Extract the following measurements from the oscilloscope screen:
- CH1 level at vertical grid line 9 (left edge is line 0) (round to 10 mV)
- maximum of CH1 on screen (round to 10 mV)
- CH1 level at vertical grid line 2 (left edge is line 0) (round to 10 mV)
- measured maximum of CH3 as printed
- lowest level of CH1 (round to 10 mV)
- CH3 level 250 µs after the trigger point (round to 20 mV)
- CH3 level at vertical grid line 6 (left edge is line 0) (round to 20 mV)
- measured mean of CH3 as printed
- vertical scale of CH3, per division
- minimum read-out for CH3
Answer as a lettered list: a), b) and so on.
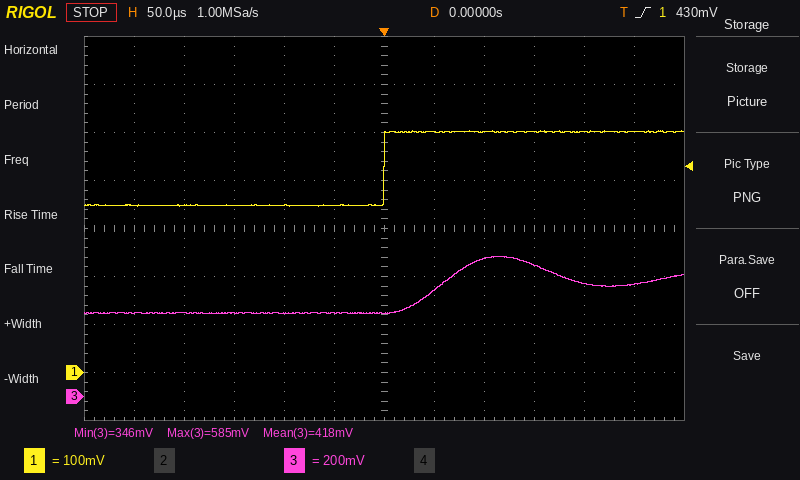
a) 500 mV
b) 500 mV
c) 350 mV
d) 585 mV
e) 350 mV
f) 460 mV
g) 340 mV
h) 418 mV
i) 200 mV
j) 346 mV
